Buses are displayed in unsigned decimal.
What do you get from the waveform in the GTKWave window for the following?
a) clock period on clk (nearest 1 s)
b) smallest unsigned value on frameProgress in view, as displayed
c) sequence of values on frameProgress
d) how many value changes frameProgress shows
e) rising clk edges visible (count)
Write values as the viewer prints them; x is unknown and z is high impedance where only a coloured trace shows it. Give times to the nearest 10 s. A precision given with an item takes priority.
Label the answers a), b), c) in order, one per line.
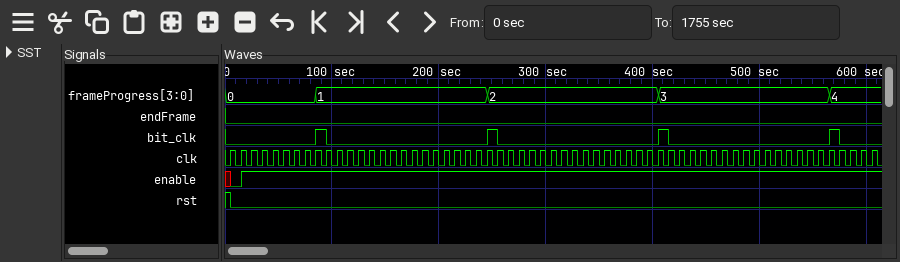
a) 10 s
b) 0
c) 0, 1, 2, 3, 4
d) 4
e) 61
